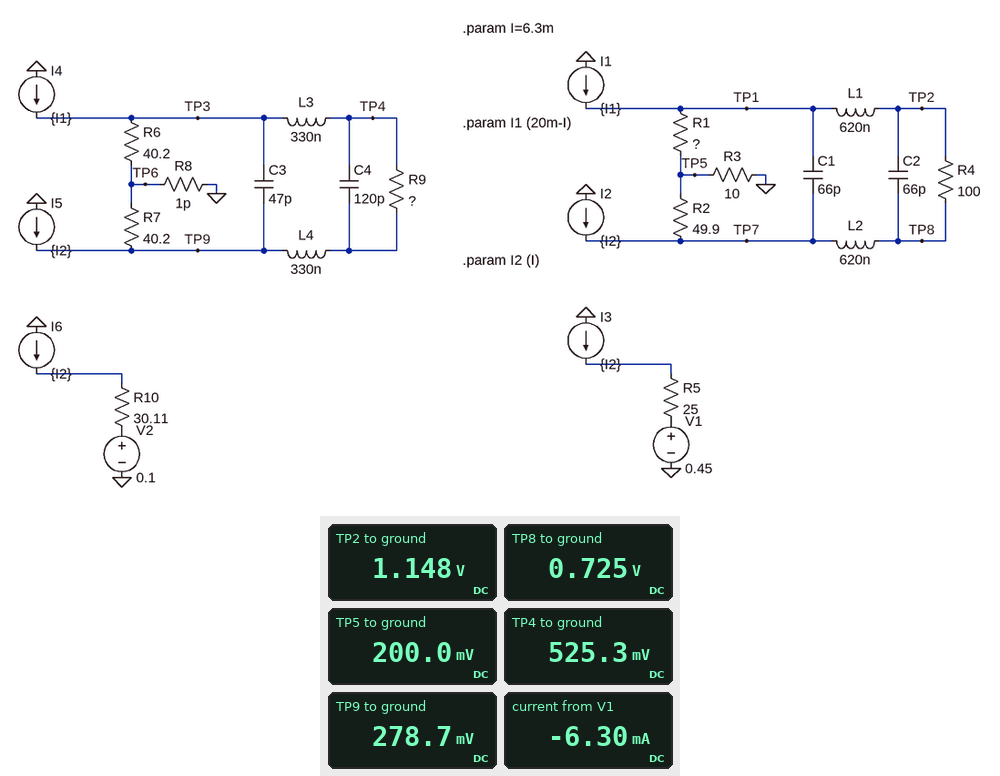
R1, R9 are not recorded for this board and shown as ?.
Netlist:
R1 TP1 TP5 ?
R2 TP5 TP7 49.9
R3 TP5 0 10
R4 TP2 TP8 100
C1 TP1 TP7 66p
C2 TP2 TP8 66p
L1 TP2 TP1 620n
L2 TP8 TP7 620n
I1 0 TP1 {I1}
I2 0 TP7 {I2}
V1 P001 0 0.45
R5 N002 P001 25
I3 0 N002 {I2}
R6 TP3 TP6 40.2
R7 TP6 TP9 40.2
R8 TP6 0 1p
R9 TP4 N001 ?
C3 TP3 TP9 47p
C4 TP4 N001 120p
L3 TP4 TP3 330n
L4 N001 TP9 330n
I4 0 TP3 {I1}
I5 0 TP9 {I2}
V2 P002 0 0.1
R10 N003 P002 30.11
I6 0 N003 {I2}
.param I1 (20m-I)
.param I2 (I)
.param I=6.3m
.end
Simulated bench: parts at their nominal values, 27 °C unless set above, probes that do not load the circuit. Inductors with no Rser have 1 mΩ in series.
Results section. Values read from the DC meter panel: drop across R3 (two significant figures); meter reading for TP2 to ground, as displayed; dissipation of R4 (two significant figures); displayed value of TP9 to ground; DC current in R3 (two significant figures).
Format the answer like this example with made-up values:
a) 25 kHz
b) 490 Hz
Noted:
a) 200 mV
b) 1.148 V
c) 1.8 mW
d) 278.7 mV
e) 20 mA
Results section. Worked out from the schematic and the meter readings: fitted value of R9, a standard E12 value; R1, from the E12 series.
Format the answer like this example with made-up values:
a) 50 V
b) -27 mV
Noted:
a) 390 Ω
b) 100 Ω
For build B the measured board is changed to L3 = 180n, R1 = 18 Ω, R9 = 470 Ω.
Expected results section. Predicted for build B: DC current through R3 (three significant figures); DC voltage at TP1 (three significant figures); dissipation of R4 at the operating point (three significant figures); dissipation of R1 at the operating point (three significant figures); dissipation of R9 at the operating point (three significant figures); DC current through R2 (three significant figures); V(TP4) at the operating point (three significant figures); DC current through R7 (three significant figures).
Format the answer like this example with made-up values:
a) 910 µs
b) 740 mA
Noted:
a) 20.0 mA
b) 454 mV
c) 16.3 µW
d) 3.58 mW
e) 137 µW
f) 5.90 mA
g) 529 mV
h) 6.84 mA
